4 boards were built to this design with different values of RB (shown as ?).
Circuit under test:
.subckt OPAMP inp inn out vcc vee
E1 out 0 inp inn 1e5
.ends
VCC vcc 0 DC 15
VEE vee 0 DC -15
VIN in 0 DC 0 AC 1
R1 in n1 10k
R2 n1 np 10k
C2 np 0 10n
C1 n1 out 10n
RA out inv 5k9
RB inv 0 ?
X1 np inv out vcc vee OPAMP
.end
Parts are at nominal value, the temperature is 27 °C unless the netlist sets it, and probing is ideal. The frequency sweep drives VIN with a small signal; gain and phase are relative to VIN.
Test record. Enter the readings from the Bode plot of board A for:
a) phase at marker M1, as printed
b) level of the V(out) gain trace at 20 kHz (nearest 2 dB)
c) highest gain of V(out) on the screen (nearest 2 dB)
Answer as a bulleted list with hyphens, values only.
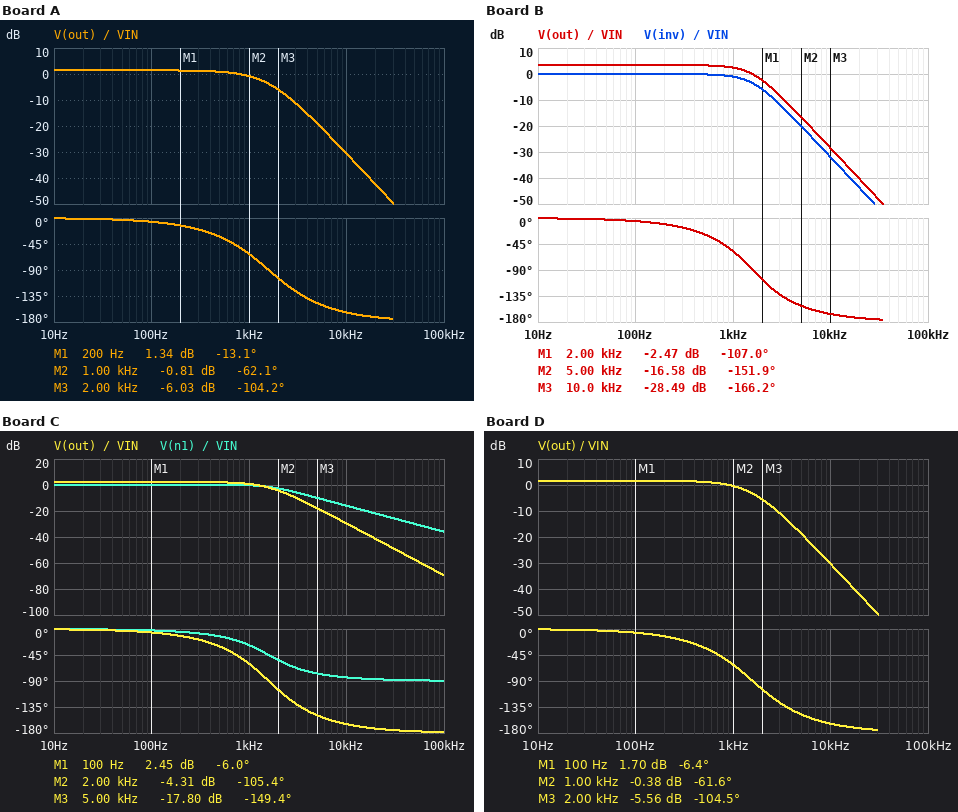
- -13.1 deg
- -42 dB
- 2 dB
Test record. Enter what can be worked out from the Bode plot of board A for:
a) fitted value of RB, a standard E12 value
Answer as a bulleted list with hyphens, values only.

- 33 kΩ
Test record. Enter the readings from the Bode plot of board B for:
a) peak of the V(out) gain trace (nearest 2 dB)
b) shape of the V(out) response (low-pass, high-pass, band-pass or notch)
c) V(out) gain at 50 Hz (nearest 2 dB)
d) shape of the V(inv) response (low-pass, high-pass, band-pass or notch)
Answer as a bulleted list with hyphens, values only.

- 4 dB
- low-pass
- 4 dB
- low-pass
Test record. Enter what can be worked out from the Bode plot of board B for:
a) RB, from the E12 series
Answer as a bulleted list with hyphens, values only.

- 12 kΩ
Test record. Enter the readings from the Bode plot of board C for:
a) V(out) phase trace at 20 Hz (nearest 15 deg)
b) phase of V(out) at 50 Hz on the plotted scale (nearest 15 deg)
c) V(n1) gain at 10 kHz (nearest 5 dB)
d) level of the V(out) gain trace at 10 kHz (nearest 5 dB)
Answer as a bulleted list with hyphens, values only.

- 0 deg
- 0 deg
- -15 dB
- -30 dB
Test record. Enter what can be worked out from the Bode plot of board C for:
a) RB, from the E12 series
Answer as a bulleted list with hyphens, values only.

- 18 kΩ
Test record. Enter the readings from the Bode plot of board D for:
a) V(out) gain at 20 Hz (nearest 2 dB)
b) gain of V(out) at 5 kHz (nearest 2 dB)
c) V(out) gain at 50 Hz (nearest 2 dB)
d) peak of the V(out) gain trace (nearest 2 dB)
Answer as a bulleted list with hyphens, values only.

- 2 dB
- -18 dB
- 2 dB
- 2 dB
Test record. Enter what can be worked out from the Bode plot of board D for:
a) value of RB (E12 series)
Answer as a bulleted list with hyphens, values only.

- 27 kΩ
